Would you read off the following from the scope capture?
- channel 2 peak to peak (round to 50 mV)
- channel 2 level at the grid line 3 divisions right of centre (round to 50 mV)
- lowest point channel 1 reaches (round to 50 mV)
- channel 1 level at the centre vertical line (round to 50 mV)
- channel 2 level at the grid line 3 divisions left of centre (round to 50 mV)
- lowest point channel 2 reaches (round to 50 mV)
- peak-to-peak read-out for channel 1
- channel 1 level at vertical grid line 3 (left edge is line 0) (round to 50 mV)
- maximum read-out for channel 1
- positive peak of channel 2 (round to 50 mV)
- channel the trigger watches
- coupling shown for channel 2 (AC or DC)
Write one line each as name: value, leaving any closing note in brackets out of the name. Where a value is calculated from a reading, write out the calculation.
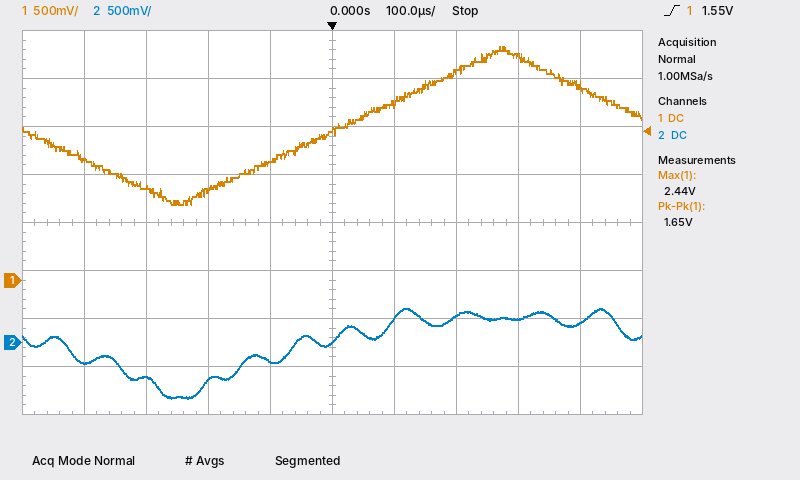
channel 2 peak to peak: 350 mV − (-600 mV) = 950 mV
channel 2 level at the grid line 3 divisions right of centre: 250 mV
lowest point channel 1 reaches: 800 mV
channel 1 level at the centre vertical line: 1.55 V
channel 2 level at the grid line 3 divisions left of centre: -350 mV
lowest point channel 2 reaches: -600 mV
peak-to-peak read-out for channel 1: 1.65 V
channel 1 level at vertical grid line 3 (left edge is line 0): 950 mV
maximum read-out for channel 1: 2.44 V
positive peak of channel 2: 350 mV
channel the trigger watches: channel 1
coupling shown for channel 2: DC
